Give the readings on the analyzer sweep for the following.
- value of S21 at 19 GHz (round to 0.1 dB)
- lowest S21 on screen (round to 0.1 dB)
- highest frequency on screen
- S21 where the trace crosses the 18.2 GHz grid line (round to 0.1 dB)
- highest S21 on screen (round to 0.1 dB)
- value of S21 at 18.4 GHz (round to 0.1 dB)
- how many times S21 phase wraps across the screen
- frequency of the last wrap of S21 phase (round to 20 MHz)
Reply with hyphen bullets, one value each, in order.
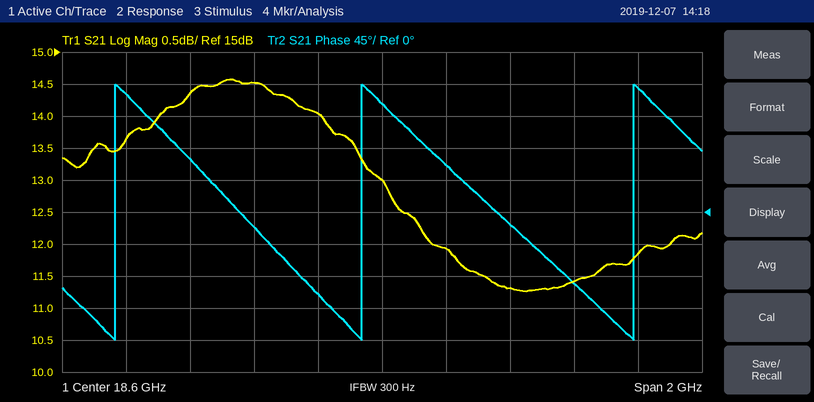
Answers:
- 11.3 dB
- 11.3 dB
- 19.6 GHz
- 14.5 dB
- 14.6 dB
- 14.0 dB
- 3
- 19.38 GHz
